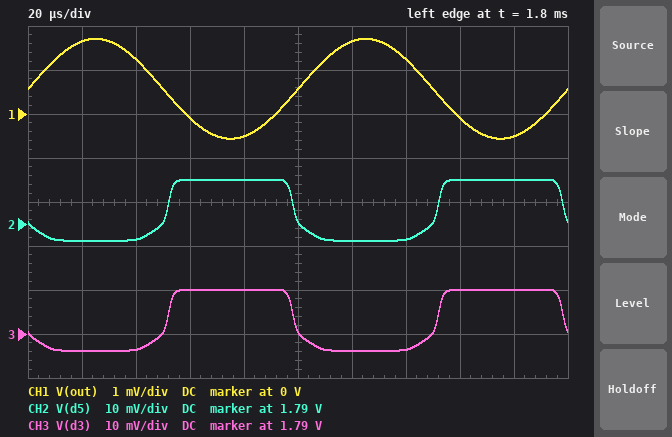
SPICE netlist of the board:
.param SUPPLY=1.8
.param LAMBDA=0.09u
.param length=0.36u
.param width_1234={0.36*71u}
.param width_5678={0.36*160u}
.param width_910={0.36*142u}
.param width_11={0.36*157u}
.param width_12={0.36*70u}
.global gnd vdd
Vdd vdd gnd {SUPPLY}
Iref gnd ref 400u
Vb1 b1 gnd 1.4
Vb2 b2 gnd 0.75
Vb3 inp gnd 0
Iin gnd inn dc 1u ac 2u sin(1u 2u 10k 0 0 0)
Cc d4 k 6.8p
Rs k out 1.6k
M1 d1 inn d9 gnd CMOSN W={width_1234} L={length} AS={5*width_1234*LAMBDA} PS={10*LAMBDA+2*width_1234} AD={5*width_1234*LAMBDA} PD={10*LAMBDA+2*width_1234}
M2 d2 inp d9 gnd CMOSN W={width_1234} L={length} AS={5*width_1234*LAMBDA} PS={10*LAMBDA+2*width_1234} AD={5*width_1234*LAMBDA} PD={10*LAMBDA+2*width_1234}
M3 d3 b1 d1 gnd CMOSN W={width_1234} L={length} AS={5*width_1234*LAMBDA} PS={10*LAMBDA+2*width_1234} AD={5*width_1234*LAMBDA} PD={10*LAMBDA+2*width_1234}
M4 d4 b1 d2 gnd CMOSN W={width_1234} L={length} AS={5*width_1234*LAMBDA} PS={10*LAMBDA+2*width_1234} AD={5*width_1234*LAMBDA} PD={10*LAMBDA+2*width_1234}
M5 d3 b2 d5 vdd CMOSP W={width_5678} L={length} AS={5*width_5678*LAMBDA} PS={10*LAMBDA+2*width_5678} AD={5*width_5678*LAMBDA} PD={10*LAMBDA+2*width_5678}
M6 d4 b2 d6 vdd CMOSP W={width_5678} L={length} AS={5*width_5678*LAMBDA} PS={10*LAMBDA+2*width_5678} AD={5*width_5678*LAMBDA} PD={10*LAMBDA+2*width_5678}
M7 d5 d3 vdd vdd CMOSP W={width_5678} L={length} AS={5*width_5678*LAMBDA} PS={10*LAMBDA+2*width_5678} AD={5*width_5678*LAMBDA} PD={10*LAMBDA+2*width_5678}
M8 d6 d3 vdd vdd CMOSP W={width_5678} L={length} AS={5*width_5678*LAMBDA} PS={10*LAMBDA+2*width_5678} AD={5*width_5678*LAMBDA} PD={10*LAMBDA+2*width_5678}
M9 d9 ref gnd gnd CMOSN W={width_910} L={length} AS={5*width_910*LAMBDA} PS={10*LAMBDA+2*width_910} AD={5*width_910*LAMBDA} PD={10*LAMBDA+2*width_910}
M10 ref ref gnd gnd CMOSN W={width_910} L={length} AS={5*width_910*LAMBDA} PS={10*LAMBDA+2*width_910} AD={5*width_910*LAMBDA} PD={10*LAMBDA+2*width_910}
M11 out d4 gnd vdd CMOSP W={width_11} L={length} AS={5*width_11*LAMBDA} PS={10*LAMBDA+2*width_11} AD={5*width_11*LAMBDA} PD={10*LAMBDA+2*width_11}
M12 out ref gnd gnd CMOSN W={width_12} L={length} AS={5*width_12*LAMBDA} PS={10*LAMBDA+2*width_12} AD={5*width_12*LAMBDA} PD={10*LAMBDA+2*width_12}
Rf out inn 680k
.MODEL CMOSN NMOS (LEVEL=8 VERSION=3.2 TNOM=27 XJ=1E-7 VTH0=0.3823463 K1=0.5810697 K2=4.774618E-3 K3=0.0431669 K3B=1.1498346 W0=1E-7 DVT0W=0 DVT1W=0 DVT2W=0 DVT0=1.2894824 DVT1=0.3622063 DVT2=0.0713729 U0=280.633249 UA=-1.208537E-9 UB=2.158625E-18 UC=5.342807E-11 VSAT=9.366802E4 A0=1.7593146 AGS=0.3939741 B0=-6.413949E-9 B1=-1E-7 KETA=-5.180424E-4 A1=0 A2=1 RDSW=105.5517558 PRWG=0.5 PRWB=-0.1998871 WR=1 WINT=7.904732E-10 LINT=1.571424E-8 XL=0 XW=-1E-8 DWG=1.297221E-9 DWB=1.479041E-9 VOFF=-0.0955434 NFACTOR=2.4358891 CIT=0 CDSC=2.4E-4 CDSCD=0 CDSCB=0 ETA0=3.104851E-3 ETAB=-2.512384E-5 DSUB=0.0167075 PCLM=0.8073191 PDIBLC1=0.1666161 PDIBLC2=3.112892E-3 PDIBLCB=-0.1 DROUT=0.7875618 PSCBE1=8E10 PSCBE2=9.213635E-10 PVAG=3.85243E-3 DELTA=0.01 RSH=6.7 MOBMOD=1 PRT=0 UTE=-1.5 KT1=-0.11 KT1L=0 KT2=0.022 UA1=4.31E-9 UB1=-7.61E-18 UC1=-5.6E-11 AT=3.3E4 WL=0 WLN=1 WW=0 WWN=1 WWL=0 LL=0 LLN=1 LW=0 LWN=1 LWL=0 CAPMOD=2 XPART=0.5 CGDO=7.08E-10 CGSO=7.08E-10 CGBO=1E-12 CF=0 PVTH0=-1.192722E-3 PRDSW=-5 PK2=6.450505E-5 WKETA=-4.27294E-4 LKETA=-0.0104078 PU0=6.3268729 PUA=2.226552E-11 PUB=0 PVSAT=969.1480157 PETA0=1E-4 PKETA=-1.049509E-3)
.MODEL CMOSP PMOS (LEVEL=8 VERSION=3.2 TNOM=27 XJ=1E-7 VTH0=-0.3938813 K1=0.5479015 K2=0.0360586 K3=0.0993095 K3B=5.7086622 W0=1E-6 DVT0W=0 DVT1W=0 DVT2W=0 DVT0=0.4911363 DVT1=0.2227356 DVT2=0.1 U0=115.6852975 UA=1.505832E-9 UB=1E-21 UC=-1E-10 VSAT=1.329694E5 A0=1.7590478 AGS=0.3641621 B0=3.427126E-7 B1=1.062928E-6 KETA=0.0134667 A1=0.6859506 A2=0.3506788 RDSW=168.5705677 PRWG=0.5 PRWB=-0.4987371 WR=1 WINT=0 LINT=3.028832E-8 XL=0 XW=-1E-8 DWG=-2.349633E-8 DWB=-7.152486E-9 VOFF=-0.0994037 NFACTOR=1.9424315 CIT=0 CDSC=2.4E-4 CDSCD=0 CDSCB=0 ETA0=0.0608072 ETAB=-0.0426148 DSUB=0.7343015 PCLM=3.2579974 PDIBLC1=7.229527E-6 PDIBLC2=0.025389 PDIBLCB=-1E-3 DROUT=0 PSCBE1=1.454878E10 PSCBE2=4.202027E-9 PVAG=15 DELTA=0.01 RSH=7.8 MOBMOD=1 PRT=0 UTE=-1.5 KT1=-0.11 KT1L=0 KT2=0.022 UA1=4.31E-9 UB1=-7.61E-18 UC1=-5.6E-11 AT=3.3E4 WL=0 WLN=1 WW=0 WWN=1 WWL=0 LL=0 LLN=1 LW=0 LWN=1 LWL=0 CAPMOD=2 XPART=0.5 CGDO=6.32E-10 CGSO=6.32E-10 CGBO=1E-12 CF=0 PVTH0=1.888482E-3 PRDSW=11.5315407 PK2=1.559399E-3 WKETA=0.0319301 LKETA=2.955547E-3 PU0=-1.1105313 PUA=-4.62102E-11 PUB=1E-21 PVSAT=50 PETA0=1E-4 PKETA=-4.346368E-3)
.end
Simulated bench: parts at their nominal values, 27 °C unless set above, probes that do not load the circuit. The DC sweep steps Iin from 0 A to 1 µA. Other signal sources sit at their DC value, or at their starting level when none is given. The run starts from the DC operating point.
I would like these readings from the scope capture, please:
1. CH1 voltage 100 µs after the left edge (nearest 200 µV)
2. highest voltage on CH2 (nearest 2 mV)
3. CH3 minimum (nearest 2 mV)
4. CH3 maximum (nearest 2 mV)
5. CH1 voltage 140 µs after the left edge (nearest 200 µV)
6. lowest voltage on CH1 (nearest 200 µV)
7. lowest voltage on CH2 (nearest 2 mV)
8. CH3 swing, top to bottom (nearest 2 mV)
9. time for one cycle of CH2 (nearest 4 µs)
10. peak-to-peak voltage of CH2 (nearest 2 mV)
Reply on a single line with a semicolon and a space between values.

600 µV; 1.800 V; 1.786 V; 1.800 V; 1.2 mV; -600 µV; 1.786 V; 14 mV; 100 µs; 14 mV
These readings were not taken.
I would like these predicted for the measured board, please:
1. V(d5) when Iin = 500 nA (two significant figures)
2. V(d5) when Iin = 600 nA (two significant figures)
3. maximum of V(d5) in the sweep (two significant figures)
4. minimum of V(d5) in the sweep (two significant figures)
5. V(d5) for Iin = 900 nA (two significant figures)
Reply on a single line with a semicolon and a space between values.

1.8 V; 1.8 V; 1.8 V; 1.8 V; 1.8 V
